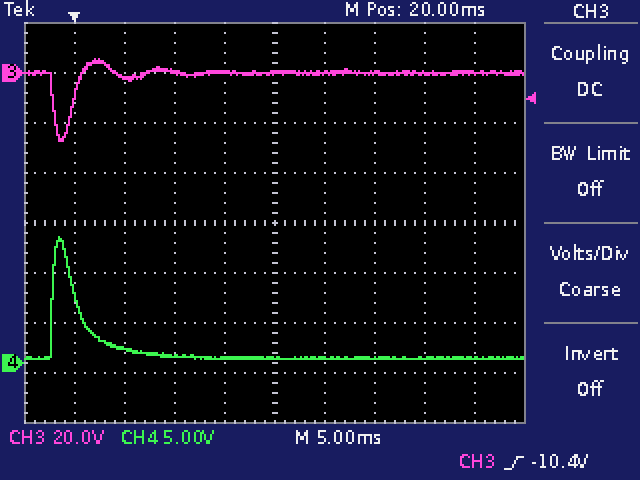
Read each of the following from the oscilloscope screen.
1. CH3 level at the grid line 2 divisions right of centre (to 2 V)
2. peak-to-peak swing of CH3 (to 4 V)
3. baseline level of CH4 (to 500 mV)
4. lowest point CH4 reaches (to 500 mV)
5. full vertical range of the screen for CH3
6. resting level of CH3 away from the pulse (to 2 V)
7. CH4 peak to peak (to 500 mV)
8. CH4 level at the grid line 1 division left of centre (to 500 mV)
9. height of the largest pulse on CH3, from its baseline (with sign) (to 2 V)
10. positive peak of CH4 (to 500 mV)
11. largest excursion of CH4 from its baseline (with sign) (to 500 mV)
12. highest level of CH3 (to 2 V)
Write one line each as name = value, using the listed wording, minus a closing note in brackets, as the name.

CH3 level at the grid line 2 divisions right of centre = 0 V
peak-to-peak swing of CH3 = 32 V
baseline level of CH4 = 500 mV
lowest point CH4 reaches = 500 mV
full vertical range of the screen for CH3 = 160 V
resting level of CH3 away from the pulse = 0 V
CH4 peak to peak = 12.0 V
CH4 level at the grid line 1 division left of centre = 500 mV
height of the largest pulse on CH3, from its baseline (with sign) = -28 V
positive peak of CH4 = 12.5 V
largest excursion of CH4 from its baseline (with sign) = +12.0 V
highest level of CH3 = 6 V
